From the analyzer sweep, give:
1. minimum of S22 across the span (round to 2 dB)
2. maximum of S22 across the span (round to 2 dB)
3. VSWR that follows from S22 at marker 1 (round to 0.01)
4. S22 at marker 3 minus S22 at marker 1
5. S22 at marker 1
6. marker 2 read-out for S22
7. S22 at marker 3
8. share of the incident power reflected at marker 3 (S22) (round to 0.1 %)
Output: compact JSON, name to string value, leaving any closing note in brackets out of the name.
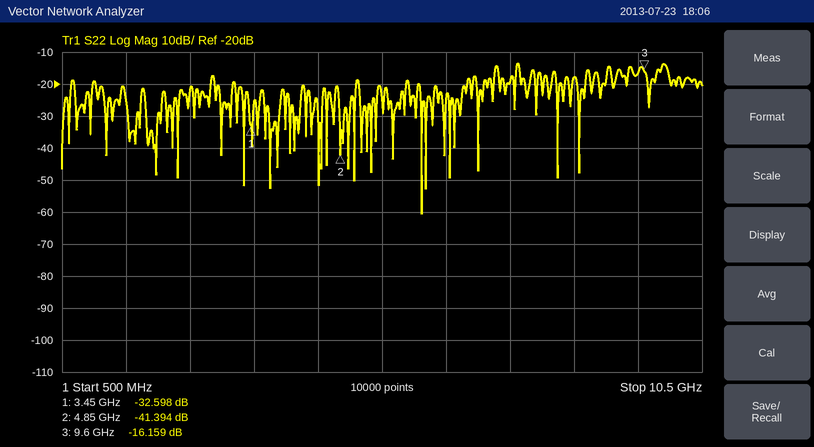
{"minimum of S22 across the span": "-60 dB", "maximum of S22 across the span": "-14 dB", "VSWR that follows from S22 at marker 1": "1.05", "S22 at marker 3 minus S22 at marker 1": "16.439 dB", "S22 at marker 1": "-32.598 dB", "marker 2 read-out for S22": "-41.394 dB", "S22 at marker 3": "-16.159 dB", "share of the incident power reflected at marker 3 (S22)": "2.4 %"}
